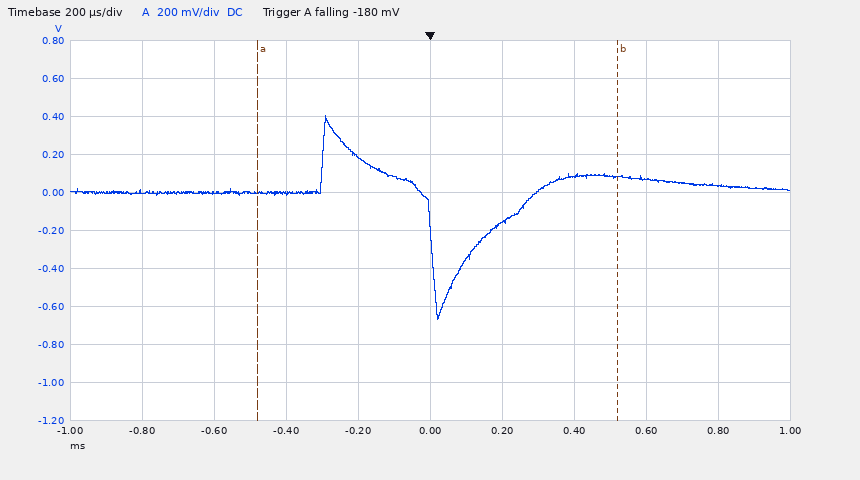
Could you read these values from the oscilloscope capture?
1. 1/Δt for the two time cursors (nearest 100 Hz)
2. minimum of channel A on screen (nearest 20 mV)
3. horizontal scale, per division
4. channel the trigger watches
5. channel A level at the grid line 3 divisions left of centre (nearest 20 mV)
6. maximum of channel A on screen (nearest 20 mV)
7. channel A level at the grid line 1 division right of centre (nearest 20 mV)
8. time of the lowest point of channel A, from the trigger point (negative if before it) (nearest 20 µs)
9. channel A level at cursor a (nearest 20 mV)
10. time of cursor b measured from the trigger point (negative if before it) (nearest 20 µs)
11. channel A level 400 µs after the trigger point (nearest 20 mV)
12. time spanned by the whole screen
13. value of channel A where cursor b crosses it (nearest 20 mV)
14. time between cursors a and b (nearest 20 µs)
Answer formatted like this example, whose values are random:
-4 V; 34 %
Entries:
1.0 kHz; -660 mV; 200 µs; channel A; 0 mV; 400 mV; -160 mV; +20 µs; 0 mV; +520 µs; 80 mV; 2 ms; 80 mV; 1.00 ms
